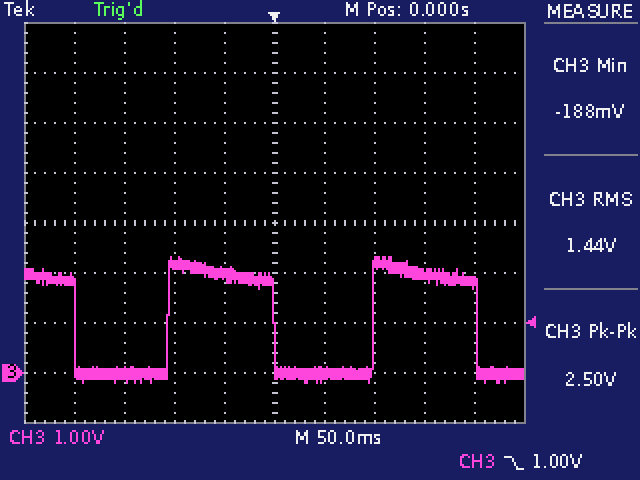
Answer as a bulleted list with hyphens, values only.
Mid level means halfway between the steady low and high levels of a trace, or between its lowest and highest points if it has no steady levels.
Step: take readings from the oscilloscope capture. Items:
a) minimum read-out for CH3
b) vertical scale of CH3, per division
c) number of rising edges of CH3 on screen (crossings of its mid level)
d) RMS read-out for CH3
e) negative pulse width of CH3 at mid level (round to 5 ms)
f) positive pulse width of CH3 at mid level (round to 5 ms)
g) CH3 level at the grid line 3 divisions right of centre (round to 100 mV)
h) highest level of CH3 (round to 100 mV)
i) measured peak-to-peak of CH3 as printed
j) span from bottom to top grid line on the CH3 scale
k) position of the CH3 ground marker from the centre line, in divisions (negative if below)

- -188 mV
- 1 V
- 2
- 1.44 V
- 95 ms
- 105 ms
- 2.0 V
- 2.3 V
- 2.50 V
- 8 V
- -3.0 div
